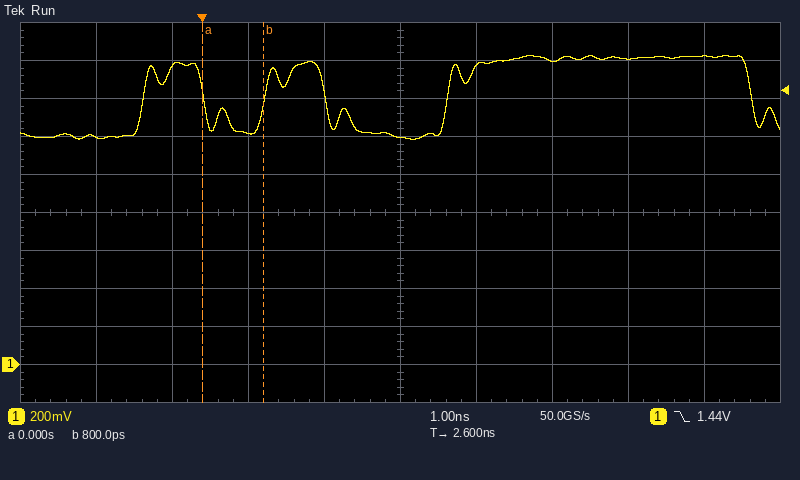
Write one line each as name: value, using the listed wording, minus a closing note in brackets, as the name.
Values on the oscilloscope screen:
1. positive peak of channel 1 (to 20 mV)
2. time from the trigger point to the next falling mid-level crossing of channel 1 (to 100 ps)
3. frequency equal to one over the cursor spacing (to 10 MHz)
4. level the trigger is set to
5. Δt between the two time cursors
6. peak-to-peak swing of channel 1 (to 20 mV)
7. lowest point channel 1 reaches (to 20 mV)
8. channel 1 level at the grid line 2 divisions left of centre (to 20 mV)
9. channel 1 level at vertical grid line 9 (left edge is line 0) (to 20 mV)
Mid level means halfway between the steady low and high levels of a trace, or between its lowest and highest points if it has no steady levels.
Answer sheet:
positive peak of channel 1: 1.62 V
time from the trigger point to the next falling mid-level crossing of channel 1: 1.6 ns
frequency equal to one over the cursor spacing: 1.25 GHz
level the trigger is set to: 1.44 V
Δt between the two time cursors: 800 ps
peak-to-peak swing of channel 1: 440 mV
lowest point channel 1 reaches: 1.18 V
channel 1 level at the grid line 2 divisions left of centre: 1.22 V
channel 1 level at vertical grid line 9 (left edge is line 0): 1.62 V
